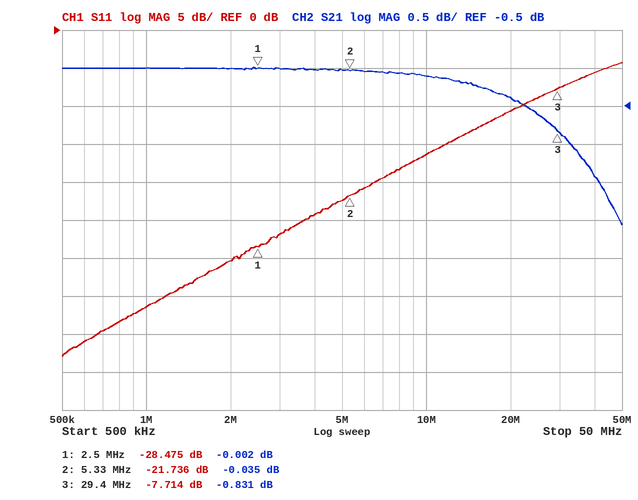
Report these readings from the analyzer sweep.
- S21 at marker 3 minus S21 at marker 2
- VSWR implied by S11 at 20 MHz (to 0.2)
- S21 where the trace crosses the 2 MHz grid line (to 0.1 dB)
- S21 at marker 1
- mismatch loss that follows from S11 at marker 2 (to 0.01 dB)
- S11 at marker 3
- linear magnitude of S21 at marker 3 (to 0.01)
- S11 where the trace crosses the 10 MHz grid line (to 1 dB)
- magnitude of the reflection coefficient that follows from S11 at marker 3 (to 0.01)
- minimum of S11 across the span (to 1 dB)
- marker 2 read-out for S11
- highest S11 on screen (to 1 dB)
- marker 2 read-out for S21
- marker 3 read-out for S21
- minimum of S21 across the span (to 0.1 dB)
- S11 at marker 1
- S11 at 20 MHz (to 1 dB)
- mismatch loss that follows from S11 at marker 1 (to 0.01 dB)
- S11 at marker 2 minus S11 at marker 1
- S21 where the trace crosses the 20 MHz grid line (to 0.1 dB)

-0.796 dB
1.8
0.0 dB
-0.002 dB
0.03 dB
-7.714 dB
0.91
-16 dB
0.41
-43 dB
-21.736 dB
-4 dB
-0.035 dB
-0.831 dB
-2.1 dB
-28.475 dB
-11 dB
0.01 dB
6.739 dB
-0.4 dB
